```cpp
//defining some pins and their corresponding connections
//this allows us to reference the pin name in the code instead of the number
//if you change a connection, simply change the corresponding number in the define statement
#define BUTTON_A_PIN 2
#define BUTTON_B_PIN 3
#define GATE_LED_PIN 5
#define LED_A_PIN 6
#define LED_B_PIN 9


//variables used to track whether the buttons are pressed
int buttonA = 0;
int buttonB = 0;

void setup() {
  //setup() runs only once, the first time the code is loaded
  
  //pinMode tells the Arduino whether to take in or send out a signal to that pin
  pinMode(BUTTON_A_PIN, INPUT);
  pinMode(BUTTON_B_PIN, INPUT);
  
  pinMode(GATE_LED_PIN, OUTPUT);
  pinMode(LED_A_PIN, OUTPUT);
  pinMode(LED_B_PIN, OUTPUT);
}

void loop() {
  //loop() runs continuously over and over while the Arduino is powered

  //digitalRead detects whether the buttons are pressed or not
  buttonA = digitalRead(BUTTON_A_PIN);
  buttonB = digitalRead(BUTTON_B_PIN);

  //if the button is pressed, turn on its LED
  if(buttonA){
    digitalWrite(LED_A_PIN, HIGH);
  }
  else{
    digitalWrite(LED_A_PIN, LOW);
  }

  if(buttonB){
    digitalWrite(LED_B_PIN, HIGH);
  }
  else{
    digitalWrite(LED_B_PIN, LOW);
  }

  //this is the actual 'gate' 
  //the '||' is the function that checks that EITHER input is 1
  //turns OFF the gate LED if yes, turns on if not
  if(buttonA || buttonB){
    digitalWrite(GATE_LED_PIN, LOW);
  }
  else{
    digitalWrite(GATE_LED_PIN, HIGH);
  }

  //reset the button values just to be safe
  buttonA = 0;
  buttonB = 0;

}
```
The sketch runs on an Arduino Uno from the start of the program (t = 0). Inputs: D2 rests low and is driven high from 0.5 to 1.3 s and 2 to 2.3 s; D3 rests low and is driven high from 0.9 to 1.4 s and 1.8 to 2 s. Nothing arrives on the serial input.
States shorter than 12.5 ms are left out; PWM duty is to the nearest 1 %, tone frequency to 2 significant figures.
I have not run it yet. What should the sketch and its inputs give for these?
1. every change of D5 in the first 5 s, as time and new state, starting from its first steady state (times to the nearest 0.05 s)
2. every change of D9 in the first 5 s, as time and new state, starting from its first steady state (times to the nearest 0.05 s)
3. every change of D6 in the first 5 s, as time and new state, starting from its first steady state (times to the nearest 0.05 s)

0 s high; 0.5 s low; 1.4 s high; 1.8 s low; 2.3 s high
0 s low; 0.9 s high; 1.4 s low; 1.8 s high; 2 s low
0 s low; 0.5 s high; 1.3 s low; 2 s high; 2.3 s low
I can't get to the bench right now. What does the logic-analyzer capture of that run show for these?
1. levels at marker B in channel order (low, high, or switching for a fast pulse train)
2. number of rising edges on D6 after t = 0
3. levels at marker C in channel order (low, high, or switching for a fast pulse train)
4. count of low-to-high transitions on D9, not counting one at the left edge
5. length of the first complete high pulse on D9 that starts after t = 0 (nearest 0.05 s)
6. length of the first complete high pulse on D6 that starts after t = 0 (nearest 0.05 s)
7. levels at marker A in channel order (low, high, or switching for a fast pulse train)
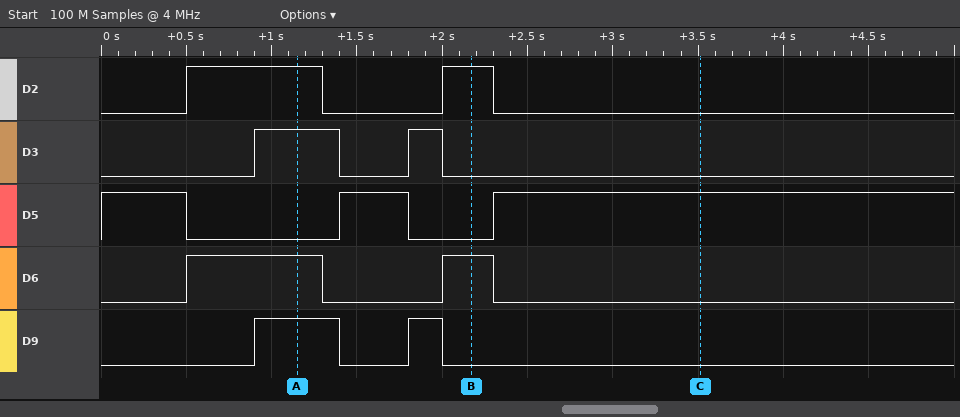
D2 high, D3 low, D5 low, D6 high, D9 low
2
D2 low, D3 low, D5 high, D6 low, D9 low
2
0.50 s
0.80 s
D2 high, D3 high, D5 low, D6 high, D9 high
